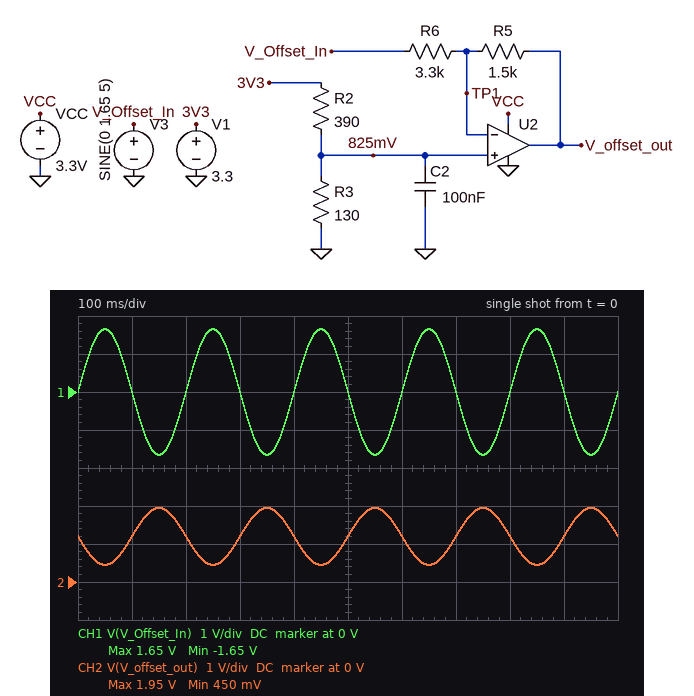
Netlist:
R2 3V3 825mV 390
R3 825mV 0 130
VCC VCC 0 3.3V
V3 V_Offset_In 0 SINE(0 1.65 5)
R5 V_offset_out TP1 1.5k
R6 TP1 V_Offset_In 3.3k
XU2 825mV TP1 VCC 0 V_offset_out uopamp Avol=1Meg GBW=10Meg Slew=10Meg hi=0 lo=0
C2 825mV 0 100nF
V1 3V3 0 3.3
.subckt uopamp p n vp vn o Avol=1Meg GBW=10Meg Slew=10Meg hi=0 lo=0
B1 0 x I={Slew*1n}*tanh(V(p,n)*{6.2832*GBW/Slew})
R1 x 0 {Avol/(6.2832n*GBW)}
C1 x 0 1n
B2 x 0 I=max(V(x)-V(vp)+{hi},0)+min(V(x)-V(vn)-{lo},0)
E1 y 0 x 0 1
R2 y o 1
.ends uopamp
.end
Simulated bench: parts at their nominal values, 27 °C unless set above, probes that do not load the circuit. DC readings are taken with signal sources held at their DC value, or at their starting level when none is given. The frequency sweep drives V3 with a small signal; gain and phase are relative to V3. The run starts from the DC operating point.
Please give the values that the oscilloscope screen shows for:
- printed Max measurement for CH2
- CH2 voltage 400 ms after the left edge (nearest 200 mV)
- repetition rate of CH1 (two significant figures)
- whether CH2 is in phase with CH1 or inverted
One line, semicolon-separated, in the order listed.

1.95 V; 1.2 V; 5.0 Hz; inverted
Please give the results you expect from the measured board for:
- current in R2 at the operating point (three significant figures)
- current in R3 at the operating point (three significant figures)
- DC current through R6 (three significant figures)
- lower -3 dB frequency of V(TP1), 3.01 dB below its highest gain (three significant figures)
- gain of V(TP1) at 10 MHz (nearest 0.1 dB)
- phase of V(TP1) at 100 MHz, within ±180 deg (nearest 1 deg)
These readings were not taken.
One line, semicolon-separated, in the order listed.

6.35 mA; 6.35 mA; 250 µA; 6.87 MHz; -11.8 dB; 4 deg
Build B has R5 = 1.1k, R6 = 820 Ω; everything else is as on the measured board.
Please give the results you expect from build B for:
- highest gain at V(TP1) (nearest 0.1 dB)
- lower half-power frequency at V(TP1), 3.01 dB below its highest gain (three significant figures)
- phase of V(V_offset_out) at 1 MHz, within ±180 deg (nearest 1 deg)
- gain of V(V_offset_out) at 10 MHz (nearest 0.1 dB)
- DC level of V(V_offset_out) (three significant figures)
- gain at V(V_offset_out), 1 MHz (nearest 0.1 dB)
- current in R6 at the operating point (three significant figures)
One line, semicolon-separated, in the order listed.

-4.8 dB; 4.27 MHz; 167 deg; -5.6 dB; 1.93 V; 2.3 dB; 1.01 mA
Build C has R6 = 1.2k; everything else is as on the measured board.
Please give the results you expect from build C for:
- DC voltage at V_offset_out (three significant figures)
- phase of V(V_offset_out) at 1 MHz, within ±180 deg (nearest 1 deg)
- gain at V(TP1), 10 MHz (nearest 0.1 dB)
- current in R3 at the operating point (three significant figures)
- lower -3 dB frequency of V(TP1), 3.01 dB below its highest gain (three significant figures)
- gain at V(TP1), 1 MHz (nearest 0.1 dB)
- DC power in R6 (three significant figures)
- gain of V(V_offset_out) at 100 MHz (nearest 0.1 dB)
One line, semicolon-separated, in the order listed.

1.86 V; 167 deg; -5.9 dB; 6.35 mA; 4.44 MHz; -18.3 dB; 567 µW; -25.1 dB
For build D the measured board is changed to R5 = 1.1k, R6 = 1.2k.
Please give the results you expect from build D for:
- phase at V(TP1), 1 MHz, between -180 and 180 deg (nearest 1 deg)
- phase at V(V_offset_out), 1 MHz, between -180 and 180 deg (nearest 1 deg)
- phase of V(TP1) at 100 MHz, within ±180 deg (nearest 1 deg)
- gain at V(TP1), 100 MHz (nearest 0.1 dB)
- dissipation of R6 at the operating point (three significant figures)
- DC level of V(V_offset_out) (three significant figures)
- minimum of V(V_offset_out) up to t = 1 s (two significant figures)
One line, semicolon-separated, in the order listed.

79 deg; 169 deg; 3 deg; -6.4 dB; 567 µW; 1.58 V; 69 mV
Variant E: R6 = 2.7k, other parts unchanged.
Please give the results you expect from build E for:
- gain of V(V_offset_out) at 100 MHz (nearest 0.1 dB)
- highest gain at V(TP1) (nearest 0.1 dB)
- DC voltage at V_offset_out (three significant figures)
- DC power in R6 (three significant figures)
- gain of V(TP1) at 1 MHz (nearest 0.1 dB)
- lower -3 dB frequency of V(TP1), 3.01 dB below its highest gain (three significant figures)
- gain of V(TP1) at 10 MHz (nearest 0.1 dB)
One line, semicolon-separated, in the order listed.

-29.0 dB; -8.9 dB; 1.28 V; 252 µW; -25.2 dB; 6.43 MHz; -10.4 dB
